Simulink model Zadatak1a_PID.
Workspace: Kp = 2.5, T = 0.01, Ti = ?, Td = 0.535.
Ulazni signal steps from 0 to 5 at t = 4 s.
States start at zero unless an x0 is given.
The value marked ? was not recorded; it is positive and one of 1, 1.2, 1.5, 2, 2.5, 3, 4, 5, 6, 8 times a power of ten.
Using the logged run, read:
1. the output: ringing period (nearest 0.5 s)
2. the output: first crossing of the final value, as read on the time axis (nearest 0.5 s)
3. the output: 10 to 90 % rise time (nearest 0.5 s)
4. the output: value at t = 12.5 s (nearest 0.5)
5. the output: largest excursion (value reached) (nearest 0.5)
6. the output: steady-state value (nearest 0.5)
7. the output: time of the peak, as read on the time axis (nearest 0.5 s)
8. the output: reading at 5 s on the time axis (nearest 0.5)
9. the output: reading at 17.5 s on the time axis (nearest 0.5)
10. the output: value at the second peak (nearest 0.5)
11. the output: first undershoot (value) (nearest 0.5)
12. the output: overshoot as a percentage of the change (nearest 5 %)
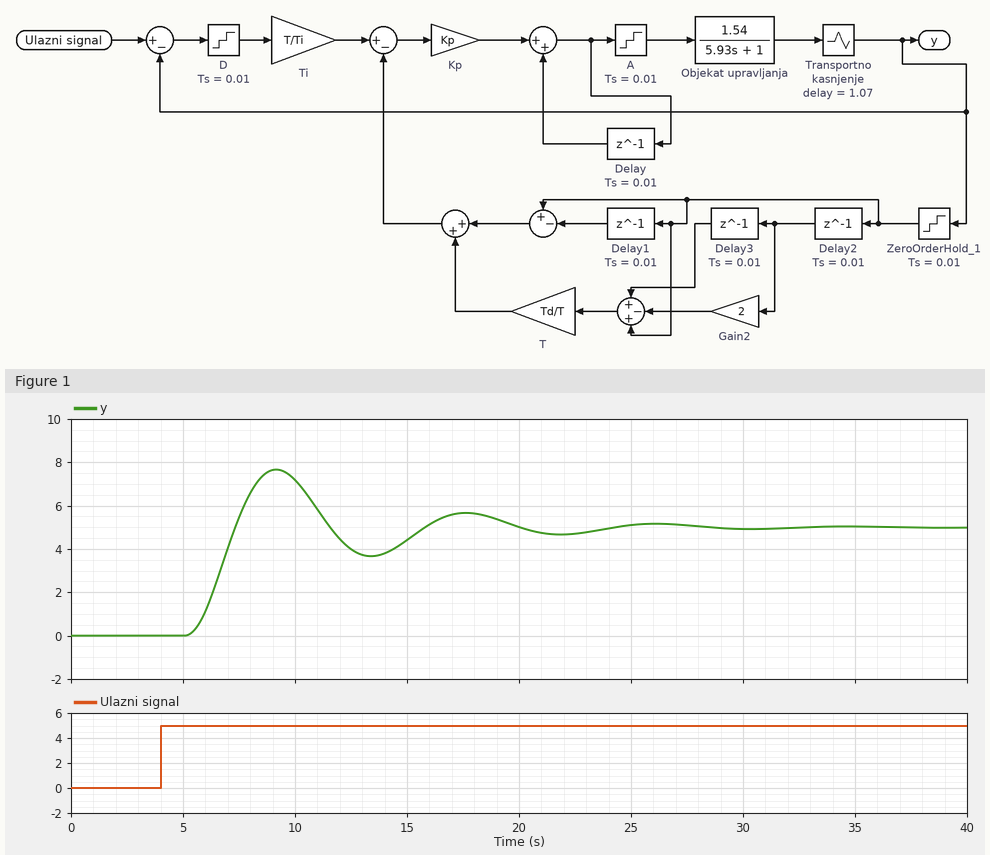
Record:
8.5 s
7.5 s
1.5 s
4.0
7.5
5.0
9.0 s
0.0
5.5
5.5
3.5
55 %
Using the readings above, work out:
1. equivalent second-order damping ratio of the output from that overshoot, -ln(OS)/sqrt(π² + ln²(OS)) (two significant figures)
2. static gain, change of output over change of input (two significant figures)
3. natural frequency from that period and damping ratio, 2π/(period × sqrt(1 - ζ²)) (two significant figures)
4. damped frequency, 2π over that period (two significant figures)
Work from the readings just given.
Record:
0.19
1.0
0.75 rad/s
0.74 rad/s
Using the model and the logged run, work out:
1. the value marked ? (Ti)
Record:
1.2
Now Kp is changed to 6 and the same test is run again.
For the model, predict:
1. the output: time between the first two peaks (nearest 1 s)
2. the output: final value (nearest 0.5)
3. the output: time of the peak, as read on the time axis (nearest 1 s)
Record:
3 s
5.0
7 s
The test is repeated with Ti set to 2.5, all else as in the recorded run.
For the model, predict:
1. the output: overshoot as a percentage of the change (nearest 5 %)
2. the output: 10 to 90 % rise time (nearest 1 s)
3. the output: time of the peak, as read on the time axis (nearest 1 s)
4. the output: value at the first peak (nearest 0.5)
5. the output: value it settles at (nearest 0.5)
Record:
10 %
3 s
12 s
5.5
5.0
